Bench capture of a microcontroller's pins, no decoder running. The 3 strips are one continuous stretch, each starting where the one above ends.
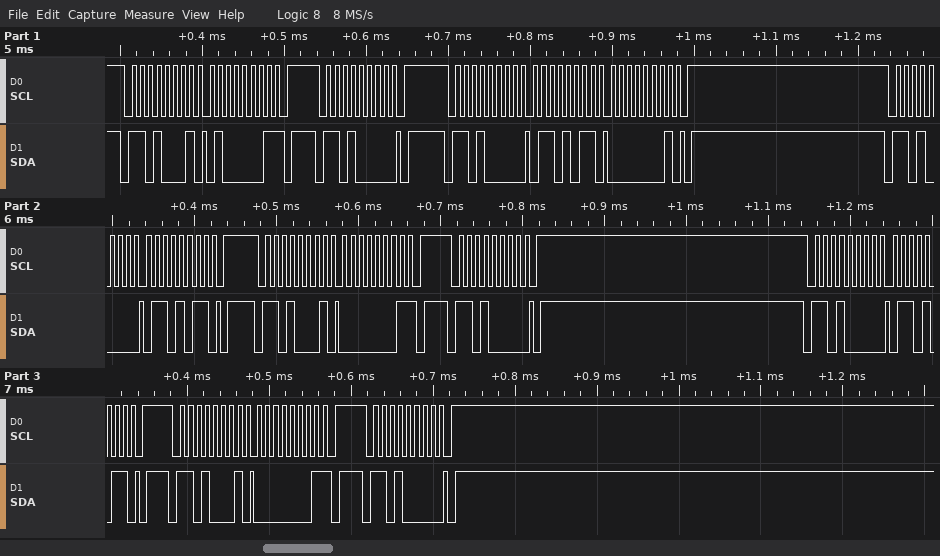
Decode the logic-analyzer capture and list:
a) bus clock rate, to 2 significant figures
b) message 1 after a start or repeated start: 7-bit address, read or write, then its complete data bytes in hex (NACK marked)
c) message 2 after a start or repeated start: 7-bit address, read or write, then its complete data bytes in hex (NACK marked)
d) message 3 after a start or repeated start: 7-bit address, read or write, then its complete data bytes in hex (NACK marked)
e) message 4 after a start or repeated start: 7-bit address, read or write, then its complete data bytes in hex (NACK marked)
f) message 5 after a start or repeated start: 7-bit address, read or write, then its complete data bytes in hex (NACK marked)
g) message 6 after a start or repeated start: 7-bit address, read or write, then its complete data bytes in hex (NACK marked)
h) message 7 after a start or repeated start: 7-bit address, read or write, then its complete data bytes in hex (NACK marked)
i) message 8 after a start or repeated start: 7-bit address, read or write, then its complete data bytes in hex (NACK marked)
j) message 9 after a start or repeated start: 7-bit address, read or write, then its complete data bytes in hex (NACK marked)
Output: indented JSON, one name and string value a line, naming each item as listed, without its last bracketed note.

{
  "bus clock rate, to 2 significant figures": "100 kHz",
  "message 1 after a start or repeated start: 7-bit address, read or write, then its complete data bytes in hex": "0x68 read: 41 NACK",
  "message 2 after a start or repeated start: 7-bit address, read or write, then its complete data bytes in hex": "0x68 write",
  "message 3 after a start or repeated start: 7-bit address, read or write, then its complete data bytes in hex": "0x68 write: 6B 01",
  "message 4 after a start or repeated start: 7-bit address, read or write, then its complete data bytes in hex": "0x68 write: 6B",
  "message 5 after a start or repeated start: 7-bit address, read or write, then its complete data bytes in hex": "0x68 read: 01 NACK",
  "message 6 after a start or repeated start: 7-bit address, read or write, then its complete data bytes in hex": "0x68 write",
  "message 7 after a start or repeated start: 7-bit address, read or write, then its complete data bytes in hex": "0x68 write: 6B",
  "message 8 after a start or repeated start: 7-bit address, read or write, then its complete data bytes in hex": "0x68 read: 01 NACK",
  "message 9 after a start or repeated start: 7-bit address, read or write, then its complete data bytes in hex": "0x68 write"
}
